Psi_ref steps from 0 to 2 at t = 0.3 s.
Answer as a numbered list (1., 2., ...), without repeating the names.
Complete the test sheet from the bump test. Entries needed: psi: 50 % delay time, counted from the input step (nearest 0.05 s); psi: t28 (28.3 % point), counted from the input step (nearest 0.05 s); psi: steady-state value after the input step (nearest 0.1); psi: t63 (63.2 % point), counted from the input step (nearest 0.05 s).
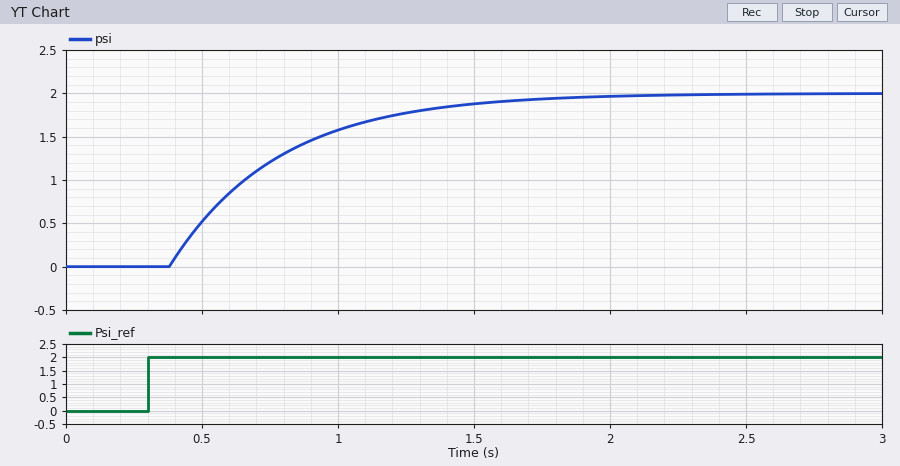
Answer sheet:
1. 0.35 s
2. 0.20 s
3. 2.0
4. 0.50 s
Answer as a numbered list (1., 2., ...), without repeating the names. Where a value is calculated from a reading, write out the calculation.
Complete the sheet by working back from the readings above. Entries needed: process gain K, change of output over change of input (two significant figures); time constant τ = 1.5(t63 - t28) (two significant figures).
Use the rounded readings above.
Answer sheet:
1. (2 - 0) / 2 = 1.0
2. 1.5 × (0.5 - 0.2) = 0.45 s
